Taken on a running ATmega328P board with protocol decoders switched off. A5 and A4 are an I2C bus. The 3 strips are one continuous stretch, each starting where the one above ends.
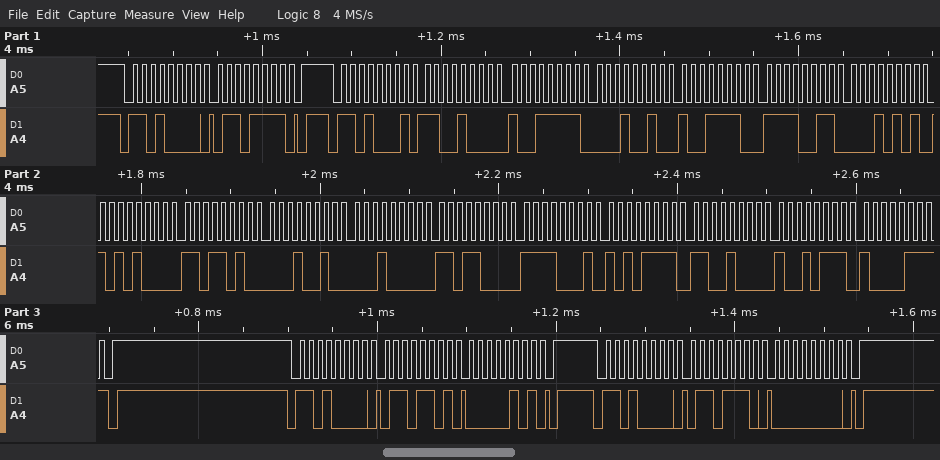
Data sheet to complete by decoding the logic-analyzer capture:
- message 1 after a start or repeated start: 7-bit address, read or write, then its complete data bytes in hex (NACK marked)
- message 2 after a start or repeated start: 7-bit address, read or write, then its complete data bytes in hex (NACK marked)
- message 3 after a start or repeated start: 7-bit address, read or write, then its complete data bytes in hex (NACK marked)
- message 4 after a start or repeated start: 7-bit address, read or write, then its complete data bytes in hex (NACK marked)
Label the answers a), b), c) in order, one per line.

a) 0x68 write: 6F
b) 0x68 read: C8 9F 12 9E F3 15 A8 DA 12 10 D8 F1 AF C8 97 87 NACK
c) 0x68 write: 6D 05
d) 0x68 write: 6E 00
